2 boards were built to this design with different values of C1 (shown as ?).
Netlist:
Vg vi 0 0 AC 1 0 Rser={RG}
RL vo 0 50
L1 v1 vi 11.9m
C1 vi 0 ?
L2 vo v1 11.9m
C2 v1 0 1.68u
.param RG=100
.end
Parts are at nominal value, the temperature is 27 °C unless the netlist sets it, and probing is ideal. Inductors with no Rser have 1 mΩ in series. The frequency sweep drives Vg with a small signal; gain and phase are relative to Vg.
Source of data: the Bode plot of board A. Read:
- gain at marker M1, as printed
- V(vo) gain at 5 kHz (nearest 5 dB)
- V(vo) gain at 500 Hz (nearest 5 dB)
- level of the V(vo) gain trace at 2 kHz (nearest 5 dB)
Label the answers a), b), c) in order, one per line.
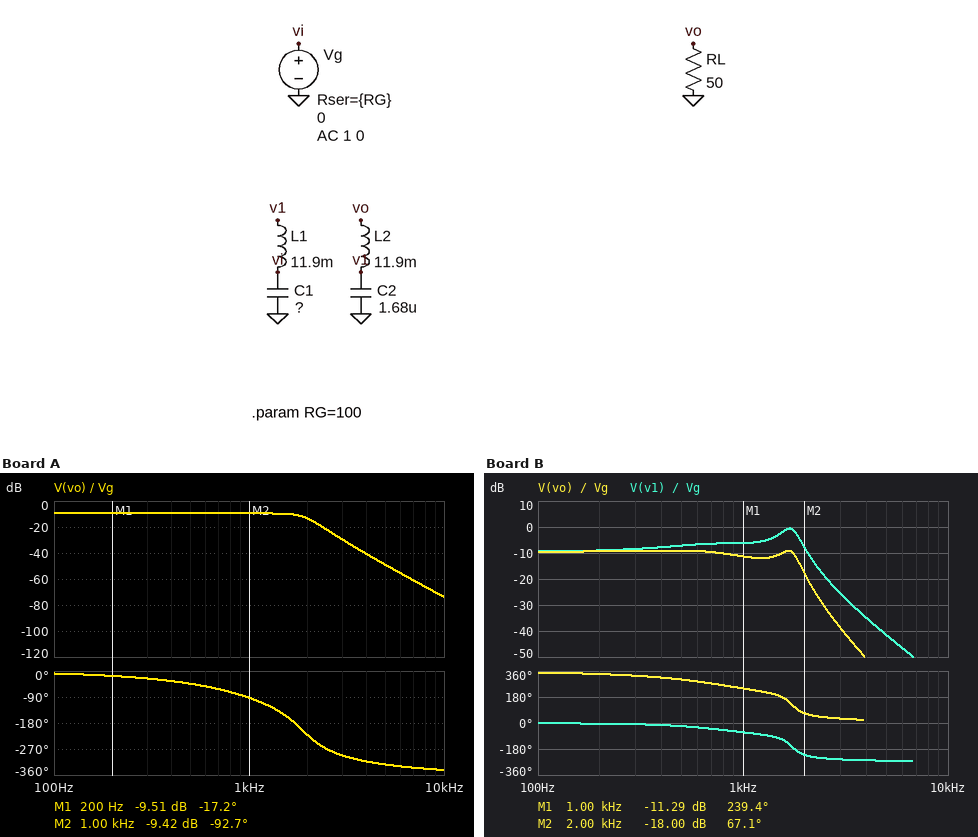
a) -9.51 dB
b) -50 dB
c) -10 dB
d) -15 dB
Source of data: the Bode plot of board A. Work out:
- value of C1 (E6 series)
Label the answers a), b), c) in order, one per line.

a) 680 nF
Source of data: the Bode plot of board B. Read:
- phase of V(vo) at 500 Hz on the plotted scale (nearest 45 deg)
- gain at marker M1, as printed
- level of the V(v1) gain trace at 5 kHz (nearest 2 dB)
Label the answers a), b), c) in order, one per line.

a) 315 deg
b) -11.29 dB
c) -42 dB
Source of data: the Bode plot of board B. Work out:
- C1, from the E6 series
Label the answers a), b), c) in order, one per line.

a) 2.2 µF
